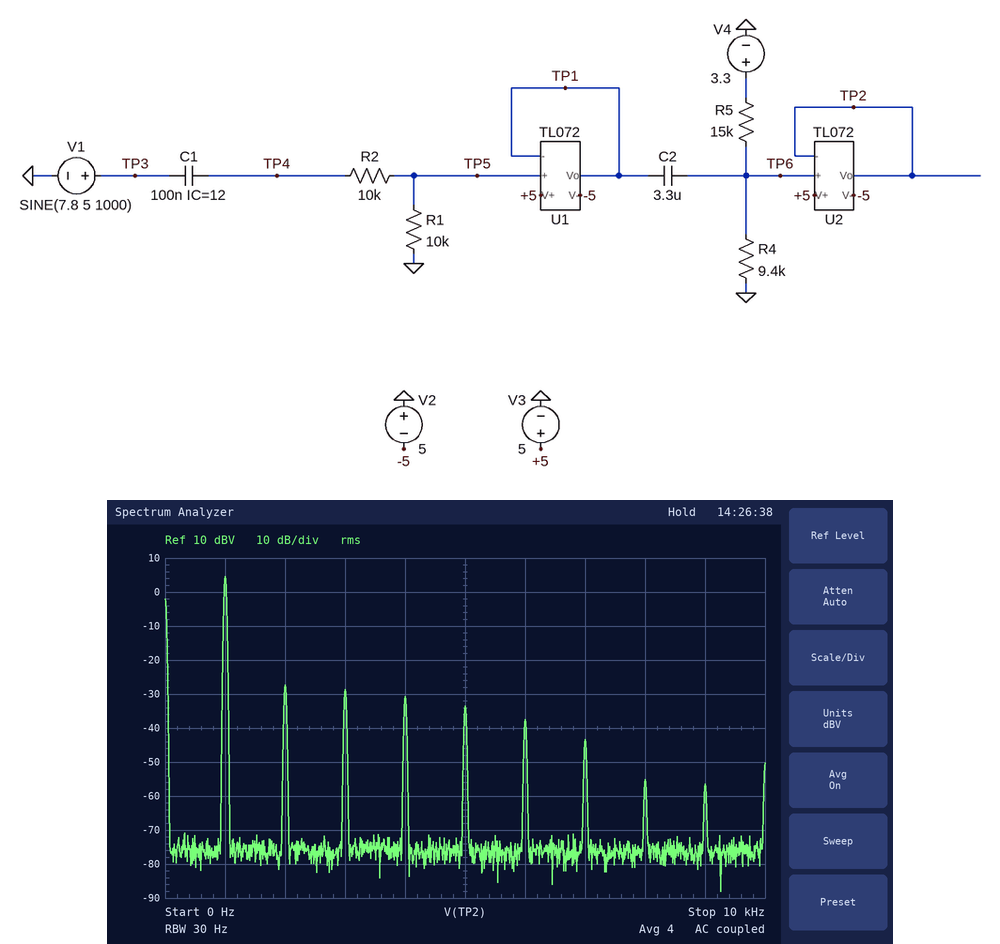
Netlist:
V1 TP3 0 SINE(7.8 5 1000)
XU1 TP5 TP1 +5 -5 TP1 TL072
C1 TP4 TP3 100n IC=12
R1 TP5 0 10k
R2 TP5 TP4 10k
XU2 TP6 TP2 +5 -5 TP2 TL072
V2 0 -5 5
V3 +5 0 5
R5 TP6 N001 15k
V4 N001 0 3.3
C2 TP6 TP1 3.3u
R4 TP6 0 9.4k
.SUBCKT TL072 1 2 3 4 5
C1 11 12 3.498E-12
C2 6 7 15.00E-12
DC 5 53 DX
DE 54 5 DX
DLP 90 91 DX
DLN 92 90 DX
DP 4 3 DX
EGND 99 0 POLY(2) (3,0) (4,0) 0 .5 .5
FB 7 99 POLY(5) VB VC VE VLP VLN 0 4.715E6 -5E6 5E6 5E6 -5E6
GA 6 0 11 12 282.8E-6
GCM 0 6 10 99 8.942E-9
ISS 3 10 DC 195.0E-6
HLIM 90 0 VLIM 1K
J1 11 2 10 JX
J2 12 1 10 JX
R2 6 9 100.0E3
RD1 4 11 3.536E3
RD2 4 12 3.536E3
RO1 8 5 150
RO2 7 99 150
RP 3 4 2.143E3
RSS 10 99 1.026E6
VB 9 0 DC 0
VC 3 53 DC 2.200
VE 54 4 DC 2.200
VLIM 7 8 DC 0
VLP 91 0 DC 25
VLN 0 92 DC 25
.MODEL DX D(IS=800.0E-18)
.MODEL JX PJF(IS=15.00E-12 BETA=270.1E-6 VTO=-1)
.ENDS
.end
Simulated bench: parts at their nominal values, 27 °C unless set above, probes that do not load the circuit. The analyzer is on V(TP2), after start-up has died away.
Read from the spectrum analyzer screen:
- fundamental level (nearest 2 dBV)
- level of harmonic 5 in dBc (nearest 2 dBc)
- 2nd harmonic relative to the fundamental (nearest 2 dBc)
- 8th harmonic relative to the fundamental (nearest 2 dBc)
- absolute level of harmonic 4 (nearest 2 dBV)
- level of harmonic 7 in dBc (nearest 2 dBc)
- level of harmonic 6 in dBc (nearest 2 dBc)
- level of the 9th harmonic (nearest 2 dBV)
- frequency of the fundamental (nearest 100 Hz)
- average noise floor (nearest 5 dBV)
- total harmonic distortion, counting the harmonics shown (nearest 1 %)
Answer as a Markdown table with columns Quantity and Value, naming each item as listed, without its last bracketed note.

| Quantity | Value |
|---|---|
| fundamental level | 4 dBV |
| level of harmonic 5 in dBc | -38 dBc |
| 2nd harmonic relative to the fundamental | -32 dBc |
| 8th harmonic relative to the fundamental | -60 dBc |
| absolute level of harmonic 4 | -30 dBV |
| level of harmonic 7 in dBc | -48 dBc |
| level of harmonic 6 in dBc | -42 dBc |
| level of the 9th harmonic | -56 dBV |
| frequency of the fundamental | 1.0 kHz |
| average noise floor | -75 dBV |
| total harmonic distortion, counting the harmonics shown | 4 % |
